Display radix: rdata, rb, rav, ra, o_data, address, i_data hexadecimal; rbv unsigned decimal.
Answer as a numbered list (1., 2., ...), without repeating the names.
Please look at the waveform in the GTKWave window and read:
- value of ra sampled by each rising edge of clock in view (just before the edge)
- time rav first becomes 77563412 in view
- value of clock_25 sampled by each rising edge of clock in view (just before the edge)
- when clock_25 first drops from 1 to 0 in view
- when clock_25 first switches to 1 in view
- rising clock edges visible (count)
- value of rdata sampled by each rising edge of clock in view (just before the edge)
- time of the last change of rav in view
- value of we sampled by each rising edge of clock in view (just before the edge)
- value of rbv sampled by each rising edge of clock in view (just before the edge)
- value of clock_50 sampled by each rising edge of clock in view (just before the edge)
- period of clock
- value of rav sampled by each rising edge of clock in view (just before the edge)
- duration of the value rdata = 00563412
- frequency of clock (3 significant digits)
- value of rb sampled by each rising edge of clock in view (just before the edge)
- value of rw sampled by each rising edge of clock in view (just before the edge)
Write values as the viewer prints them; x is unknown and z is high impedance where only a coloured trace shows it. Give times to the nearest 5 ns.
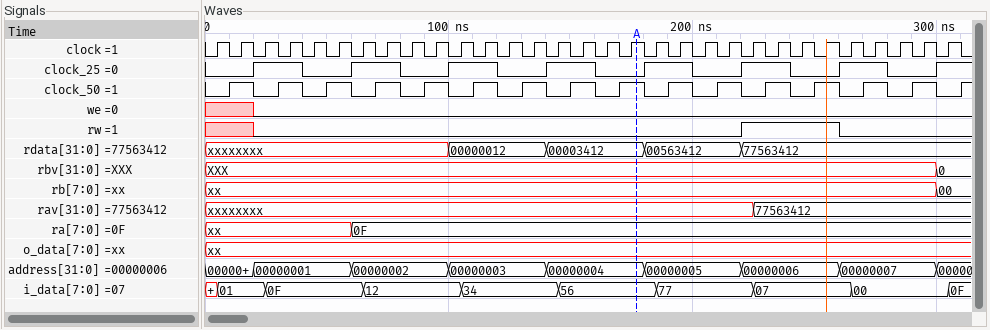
1. xx, xx, xx, xx, xx, xx, 0F, 0F, 0F, 0F, 0F, 0F, 0F, 0F, 0F, 0F, 0F, 0F, 0F, 0F, 0F, 0F, 0F, 0F, 0F, 0F, 0F, 0F, 0F, 0F, 0F
2. 225 ns
3. 0 0 1 1 0 0 1 1 0 0 1 1 0 0 1 1 0 0 1 1 0 0 1 1 0 0 1 1 0 0 1
4. 40 ns
5. 20 ns
6. 31
7. xxxxxxxx, xxxxxxxx, xxxxxxxx, xxxxxxxx, xxxxxxxx, xxxxxxxx, xxxxxxxx, xxxxxxxx, xxxxxxxx, xxxxxxxx, 00000012, 00000012, 00000012, 00000012, 00003412, 00003412, 00003412, 00003412, 00563412, 00563412, 00563412, 00563412, 77563412, 77563412, 77563412, 77563412, 77563412, 77563412, 77563412, 77563412, 77563412
8. 225 ns
9. x x 0 0 0 0 0 0 0 0 0 0 0 0 0 0 0 0 0 0 0 0 0 0 0 0 0 0 0 0 0
10. XXX, XXX, XXX, XXX, XXX, XXX, XXX, XXX, XXX, XXX, XXX, XXX, XXX, XXX, XXX, XXX, XXX, XXX, XXX, XXX, XXX, XXX, XXX, XXX, XXX, XXX, XXX, XXX, XXX, XXX, 0
11. 0 1 0 1 0 1 0 1 0 1 0 1 0 1 0 1 0 1 0 1 0 1 0 1 0 1 0 1 0 1 0
12. 10 ns
13. xxxxxxxx, xxxxxxxx, xxxxxxxx, xxxxxxxx, xxxxxxxx, xxxxxxxx, xxxxxxxx, xxxxxxxx, xxxxxxxx, xxxxxxxx, xxxxxxxx, xxxxxxxx, xxxxxxxx, xxxxxxxx, xxxxxxxx, xxxxxxxx, xxxxxxxx, xxxxxxxx, xxxxxxxx, xxxxxxxx, xxxxxxxx, xxxxxxxx, xxxxxxxx, 77563412, 77563412, 77563412, 77563412, 77563412, 77563412, 77563412, 77563412
14. 40 ns
15. 100 MHz
16. xx, xx, xx, xx, xx, xx, xx, xx, xx, xx, xx, xx, xx, xx, xx, xx, xx, xx, xx, xx, xx, xx, xx, xx, xx, xx, xx, xx, xx, xx, 00
17. x x 0 0 0 0 0 0 0 0 0 0 0 0 0 0 0 0 0 0 0 0 1 1 1 1 0 0 0 0 0
